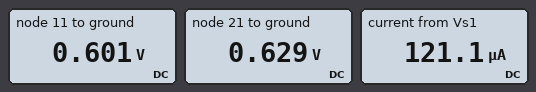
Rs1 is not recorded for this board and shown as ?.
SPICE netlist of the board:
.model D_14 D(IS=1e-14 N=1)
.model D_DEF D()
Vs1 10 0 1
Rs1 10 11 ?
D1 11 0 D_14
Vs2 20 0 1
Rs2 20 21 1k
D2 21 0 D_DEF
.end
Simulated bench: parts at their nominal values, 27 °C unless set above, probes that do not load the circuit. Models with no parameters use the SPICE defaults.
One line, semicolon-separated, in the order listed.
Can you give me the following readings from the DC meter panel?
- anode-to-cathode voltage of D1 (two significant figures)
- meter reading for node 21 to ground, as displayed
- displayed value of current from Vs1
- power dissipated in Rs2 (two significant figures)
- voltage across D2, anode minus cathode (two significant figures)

600 mV; 0.629 V; 121.1 µA; 140 µW; 630 mV
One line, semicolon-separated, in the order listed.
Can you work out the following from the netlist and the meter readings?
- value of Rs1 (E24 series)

3.3 kΩ
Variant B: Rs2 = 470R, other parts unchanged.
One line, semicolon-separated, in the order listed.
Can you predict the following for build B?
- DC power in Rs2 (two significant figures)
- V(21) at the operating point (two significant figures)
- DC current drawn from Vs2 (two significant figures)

260 µW; 650 mV; 750 µA
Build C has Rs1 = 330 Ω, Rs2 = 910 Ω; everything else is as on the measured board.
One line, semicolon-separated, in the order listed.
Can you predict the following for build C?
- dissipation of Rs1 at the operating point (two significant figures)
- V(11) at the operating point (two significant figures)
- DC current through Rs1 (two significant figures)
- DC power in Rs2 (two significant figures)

360 µW; 660 mV; 1.0 mA; 150 µW
